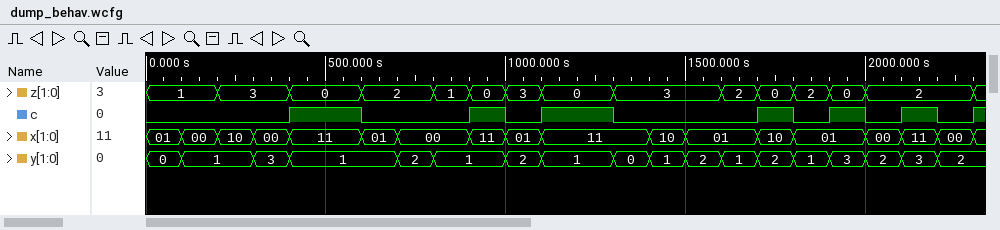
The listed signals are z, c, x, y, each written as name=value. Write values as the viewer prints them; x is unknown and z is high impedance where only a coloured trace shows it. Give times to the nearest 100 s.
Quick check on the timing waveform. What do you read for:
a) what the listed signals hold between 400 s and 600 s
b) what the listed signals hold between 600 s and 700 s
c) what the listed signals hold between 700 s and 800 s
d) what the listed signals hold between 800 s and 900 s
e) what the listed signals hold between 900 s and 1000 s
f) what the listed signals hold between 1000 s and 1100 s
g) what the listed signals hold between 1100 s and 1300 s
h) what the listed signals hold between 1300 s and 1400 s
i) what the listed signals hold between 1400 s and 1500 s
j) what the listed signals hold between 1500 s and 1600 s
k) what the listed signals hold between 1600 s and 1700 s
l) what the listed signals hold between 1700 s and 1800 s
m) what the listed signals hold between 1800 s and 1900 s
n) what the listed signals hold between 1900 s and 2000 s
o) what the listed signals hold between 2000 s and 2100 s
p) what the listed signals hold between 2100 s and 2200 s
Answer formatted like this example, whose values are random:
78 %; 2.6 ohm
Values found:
z=0, c=1, x=11, y=1; z=2, c=0, x=01, y=1; z=2, c=0, x=00, y=2; z=1, c=0, x=00, y=1; z=0, c=1, x=11, y=1; z=3, c=0, x=01, y=2; z=0, c=1, x=11, y=1; z=3, c=0, x=11, y=0; z=3, c=0, x=10, y=1; z=3, c=0, x=01, y=2; z=2, c=0, x=01, y=1; z=0, c=1, x=10, y=2; z=2, c=0, x=01, y=1; z=0, c=1, x=01, y=3; z=2, c=0, x=00, y=2; z=2, c=1, x=11, y=3
